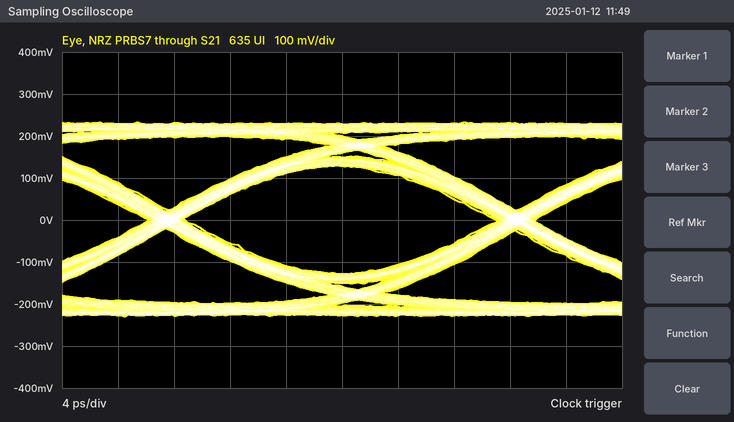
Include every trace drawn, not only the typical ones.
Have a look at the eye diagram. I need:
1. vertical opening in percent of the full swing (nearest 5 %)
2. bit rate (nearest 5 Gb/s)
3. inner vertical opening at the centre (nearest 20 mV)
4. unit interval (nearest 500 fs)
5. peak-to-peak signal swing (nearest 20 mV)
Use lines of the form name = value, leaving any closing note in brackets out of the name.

vertical opening in percent of the full swing = 55 %
bit rate = 40 Gb/s
inner vertical opening at the centre = 260 mV
unit interval = 25.0 ps
peak-to-peak signal swing = 460 mV
